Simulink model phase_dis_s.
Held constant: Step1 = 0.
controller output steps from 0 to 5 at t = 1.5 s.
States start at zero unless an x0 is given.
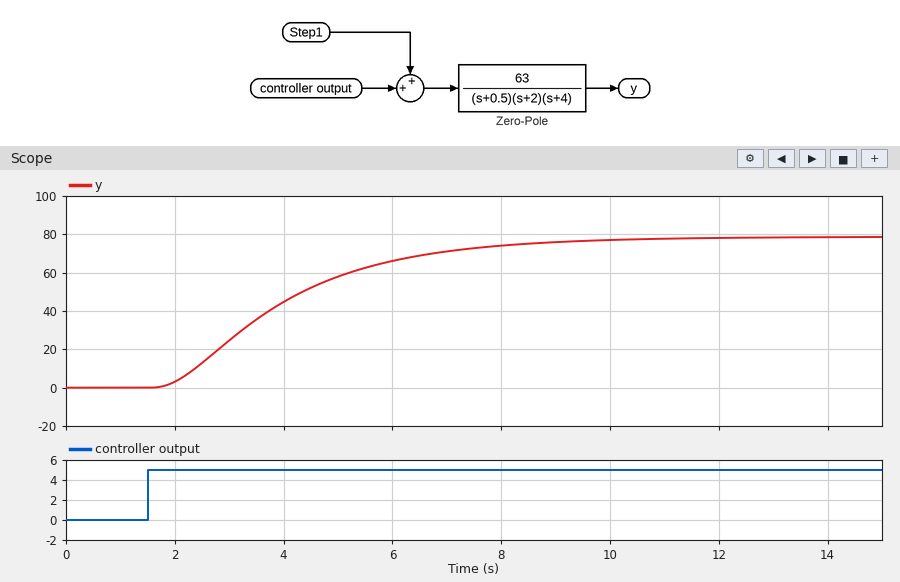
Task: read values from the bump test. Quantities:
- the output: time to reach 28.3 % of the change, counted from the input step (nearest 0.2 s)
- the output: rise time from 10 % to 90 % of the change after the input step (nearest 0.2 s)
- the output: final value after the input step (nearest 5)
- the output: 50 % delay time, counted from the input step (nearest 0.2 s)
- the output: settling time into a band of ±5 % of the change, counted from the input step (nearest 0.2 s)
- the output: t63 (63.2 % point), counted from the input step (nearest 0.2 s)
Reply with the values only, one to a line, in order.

1.4 s
4.6 s
80
2.2 s
6.8 s
2.8 s
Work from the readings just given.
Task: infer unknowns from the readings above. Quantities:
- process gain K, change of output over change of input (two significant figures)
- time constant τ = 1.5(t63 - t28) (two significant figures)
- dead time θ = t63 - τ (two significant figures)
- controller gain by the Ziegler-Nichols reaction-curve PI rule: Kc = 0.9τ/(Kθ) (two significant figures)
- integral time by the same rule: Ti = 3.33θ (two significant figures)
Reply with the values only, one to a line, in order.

16
2.1 s
0.70 s
0.17
2.3 s
